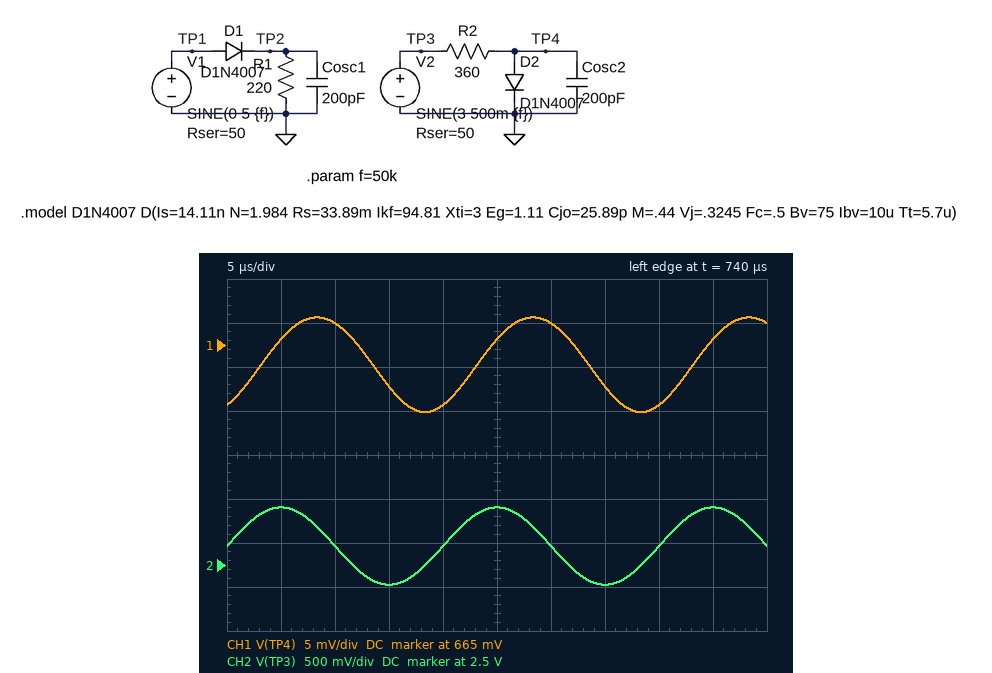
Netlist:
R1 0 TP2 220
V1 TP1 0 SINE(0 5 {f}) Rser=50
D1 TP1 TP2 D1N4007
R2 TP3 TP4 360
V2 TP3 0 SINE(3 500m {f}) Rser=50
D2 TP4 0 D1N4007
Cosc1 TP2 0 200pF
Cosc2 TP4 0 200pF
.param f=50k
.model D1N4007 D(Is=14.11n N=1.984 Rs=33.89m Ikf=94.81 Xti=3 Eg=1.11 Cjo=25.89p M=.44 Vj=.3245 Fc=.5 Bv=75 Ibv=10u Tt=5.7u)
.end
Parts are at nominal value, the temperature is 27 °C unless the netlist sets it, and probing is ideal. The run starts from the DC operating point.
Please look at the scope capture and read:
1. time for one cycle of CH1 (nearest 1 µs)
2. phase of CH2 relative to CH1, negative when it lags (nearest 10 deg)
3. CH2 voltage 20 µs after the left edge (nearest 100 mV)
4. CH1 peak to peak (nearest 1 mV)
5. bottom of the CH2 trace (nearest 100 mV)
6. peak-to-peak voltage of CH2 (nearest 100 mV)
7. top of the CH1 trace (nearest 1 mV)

20 µs
60 deg
2.7 V
11 mV
2.3 V
900 mV
668 mV
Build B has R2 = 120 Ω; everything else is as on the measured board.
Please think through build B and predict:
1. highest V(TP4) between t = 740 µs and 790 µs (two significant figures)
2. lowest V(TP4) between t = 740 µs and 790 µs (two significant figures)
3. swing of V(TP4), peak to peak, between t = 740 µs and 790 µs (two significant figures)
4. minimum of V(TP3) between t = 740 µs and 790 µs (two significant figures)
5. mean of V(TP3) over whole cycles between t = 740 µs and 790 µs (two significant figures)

710 mV
700 mV
11 mV
2.0 V
2.3 V
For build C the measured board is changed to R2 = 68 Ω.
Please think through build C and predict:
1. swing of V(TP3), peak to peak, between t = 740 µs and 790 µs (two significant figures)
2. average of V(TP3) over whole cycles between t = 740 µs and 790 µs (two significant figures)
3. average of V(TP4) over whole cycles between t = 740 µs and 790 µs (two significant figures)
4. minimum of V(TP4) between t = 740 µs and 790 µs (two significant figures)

580 mV
2.0 V
730 mV
720 mV
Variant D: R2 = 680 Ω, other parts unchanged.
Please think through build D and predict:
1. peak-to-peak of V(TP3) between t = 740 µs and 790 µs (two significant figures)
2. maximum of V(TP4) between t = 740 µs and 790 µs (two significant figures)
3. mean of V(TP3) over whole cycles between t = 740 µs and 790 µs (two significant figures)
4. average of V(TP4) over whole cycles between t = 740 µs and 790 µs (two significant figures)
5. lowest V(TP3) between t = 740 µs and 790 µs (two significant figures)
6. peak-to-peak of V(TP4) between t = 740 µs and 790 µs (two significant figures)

930 mV
640 mV
2.8 V
630 mV
2.4 V
11 mV
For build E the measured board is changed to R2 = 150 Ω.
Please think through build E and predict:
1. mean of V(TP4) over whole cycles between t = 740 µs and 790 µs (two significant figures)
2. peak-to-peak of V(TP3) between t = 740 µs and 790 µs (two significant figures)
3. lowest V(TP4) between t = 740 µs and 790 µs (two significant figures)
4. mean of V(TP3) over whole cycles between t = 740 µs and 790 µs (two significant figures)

700 mV
750 mV
690 mV
2.4 V
